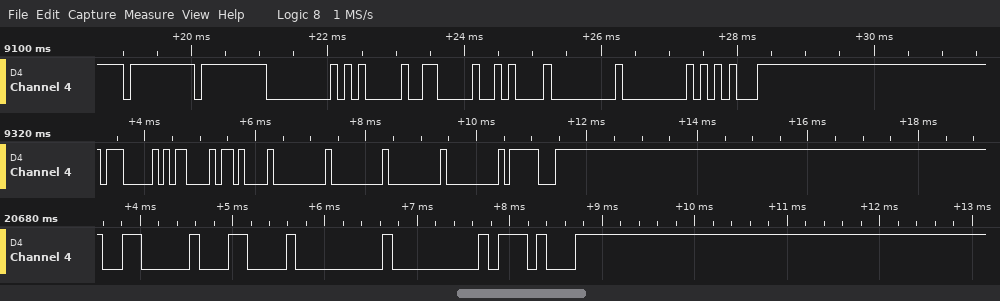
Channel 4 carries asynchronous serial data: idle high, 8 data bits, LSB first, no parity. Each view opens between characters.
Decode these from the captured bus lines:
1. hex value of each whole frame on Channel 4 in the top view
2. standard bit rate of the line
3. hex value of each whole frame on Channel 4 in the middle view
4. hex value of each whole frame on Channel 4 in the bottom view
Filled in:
FF, FF, 00, 05, 06, 0A, 00, 00, 15
9600 baud
07, 0D, 0B, 00, 00, 00, 00, 1F
06, 0C, 00, 00, 17
